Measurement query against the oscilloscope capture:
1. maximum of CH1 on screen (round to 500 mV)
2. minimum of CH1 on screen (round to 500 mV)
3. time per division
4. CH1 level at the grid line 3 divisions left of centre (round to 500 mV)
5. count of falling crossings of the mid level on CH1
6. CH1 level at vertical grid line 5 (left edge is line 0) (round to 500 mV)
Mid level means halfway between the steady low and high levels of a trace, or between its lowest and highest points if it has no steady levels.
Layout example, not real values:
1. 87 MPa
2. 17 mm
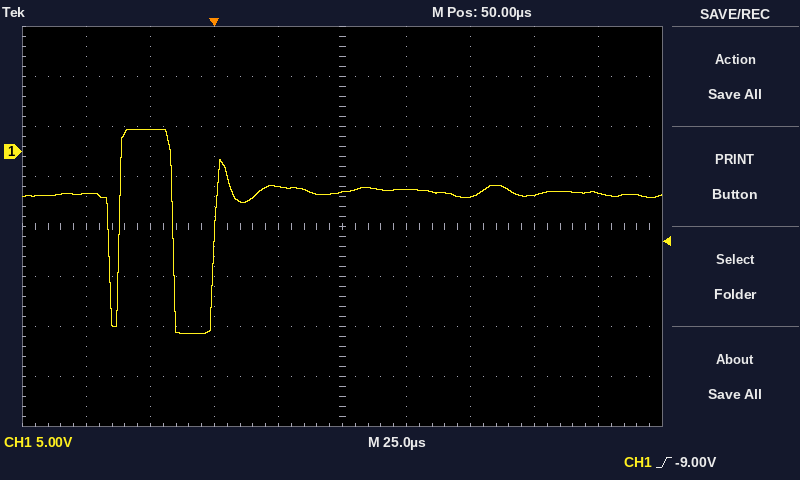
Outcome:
1. 2.0 V
2. -18.0 V
3. 25 µs
4. 2.0 V
5. 2
6. -4.0 V
